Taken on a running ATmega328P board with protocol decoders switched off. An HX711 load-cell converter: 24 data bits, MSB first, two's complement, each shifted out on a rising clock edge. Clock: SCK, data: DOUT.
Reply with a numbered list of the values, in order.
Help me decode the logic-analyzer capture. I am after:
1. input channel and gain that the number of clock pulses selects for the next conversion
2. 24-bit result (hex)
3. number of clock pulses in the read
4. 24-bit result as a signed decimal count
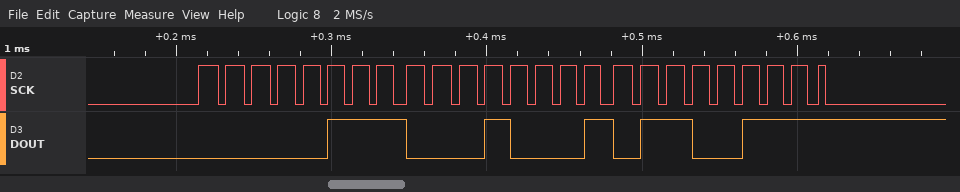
1. channel A, gain 128
2. 0x071167
3. 25
4. 463207
